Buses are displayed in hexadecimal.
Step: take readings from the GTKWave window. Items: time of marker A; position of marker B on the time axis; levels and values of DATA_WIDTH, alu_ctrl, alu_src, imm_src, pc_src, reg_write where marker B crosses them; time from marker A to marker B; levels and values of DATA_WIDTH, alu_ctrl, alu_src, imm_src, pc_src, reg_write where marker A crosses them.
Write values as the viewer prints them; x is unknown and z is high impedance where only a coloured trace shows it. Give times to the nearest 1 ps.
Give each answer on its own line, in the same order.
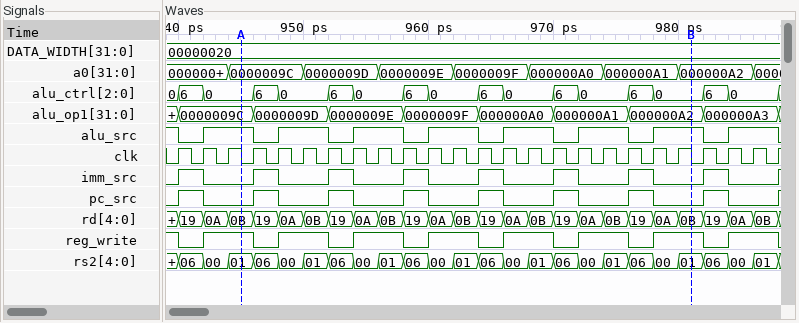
945 ps
981 ps
DATA_WIDTH=00000020, alu_ctrl=0, alu_src=1, imm_src=0, pc_src=0, reg_write=1
36 ps
DATA_WIDTH=00000020, alu_ctrl=0, alu_src=1, imm_src=0, pc_src=0, reg_write=1
